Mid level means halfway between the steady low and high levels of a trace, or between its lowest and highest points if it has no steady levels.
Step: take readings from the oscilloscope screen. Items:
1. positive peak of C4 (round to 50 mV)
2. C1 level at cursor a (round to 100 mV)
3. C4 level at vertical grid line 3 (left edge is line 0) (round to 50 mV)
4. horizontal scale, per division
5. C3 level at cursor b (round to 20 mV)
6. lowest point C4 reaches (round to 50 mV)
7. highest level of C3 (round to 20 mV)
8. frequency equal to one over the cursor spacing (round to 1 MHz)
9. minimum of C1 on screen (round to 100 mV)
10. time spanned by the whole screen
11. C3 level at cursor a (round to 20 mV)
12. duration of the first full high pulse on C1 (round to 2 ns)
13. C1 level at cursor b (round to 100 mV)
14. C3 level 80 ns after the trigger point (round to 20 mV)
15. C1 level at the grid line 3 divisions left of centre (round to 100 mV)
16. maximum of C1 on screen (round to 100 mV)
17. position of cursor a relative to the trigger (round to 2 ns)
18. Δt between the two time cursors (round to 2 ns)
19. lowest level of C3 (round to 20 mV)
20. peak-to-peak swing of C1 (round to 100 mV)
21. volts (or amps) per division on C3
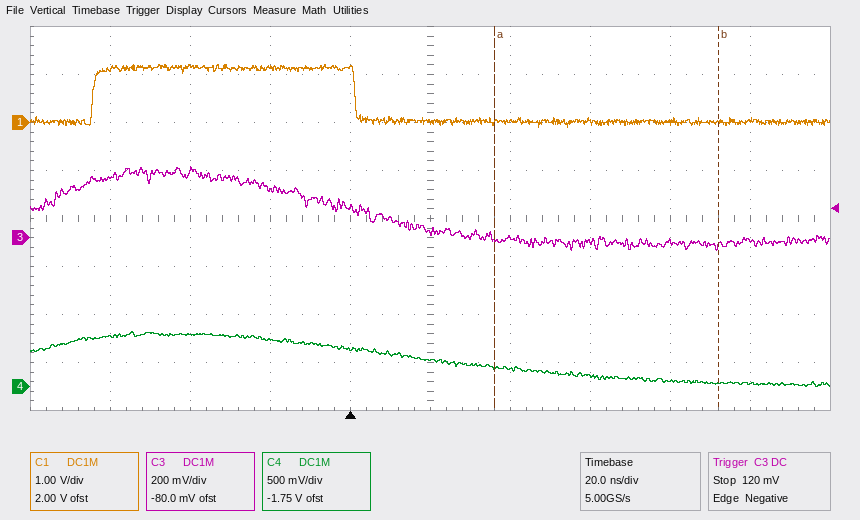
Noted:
550 mV
0.0 V
500 mV
20 ns
-40 mV
0 mV
300 mV
18 MHz
-100 mV
200 ns
0 mV
66 ns
0.0 V
-20 mV
1.2 V
1.2 V
+36 ns
56 ns
-60 mV
1.3 V
200 mV
